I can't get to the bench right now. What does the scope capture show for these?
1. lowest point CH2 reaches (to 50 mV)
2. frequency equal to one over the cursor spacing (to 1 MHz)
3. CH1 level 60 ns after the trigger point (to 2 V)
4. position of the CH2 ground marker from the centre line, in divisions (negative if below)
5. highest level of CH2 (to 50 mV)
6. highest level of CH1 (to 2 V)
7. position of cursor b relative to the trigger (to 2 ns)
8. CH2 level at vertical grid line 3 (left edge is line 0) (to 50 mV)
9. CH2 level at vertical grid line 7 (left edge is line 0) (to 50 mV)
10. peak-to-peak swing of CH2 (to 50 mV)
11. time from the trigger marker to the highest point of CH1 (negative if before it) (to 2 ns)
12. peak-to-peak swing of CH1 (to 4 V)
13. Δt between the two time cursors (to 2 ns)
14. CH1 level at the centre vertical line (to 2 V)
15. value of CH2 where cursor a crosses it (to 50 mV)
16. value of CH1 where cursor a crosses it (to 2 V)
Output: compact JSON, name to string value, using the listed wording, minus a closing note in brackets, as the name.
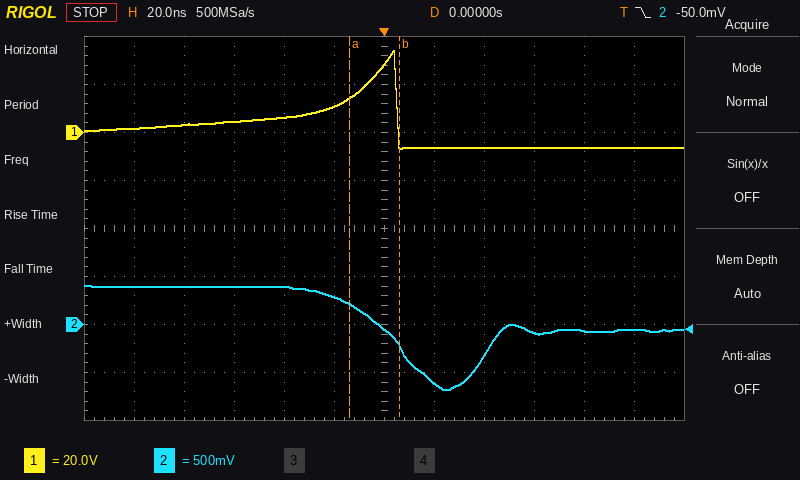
{"lowest point CH2 reaches": "-700 mV", "frequency equal to one over the cursor spacing": "50 MHz", "CH1 level 60 ns after the trigger point": "-6 V", "position of the CH2 ground marker from the centre line, in divisions": "-2.0 div", "highest level of CH2": "400 mV", "highest level of CH1": "34 V", "position of cursor b relative to the trigger": "+6 ns", "CH2 level at vertical grid line 3 (left edge is line 0)": "400 mV", "CH2 level at vertical grid line 7 (left edge is line 0)": "-600 mV", "peak-to-peak swing of CH2": "1.10 V", "time from the trigger marker to the highest point of CH1 (negative if before it)": "+4 ns", "peak-to-peak swing of CH1": "40 V", "Δt between the two time cursors": "20 ns", "CH1 level at the centre vertical line": "28 V", "value of CH2 where cursor a crosses it": "200 mV", "value of CH1 where cursor a crosses it": "14 V"}
